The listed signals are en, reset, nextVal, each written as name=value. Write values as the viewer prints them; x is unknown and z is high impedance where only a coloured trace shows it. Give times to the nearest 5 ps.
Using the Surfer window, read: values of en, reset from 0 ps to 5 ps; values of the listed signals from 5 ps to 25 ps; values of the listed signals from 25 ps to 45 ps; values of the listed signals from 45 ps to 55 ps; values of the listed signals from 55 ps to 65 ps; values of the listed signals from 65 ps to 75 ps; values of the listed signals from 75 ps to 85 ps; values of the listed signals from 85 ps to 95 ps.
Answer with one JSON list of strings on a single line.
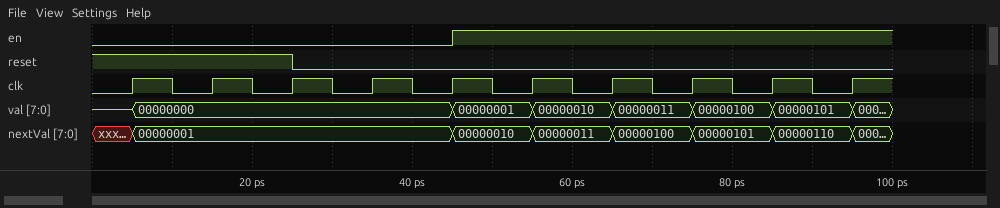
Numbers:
["en=0, reset=1", "en=0, reset=1, nextVal=00000001", "en=0, reset=0, nextVal=00000001", "en=1, reset=0, nextVal=00000010", "en=1, reset=0, nextVal=00000011", "en=1, reset=0, nextVal=00000100", "en=1, reset=0, nextVal=00000101", "en=1, reset=0, nextVal=00000110"]
